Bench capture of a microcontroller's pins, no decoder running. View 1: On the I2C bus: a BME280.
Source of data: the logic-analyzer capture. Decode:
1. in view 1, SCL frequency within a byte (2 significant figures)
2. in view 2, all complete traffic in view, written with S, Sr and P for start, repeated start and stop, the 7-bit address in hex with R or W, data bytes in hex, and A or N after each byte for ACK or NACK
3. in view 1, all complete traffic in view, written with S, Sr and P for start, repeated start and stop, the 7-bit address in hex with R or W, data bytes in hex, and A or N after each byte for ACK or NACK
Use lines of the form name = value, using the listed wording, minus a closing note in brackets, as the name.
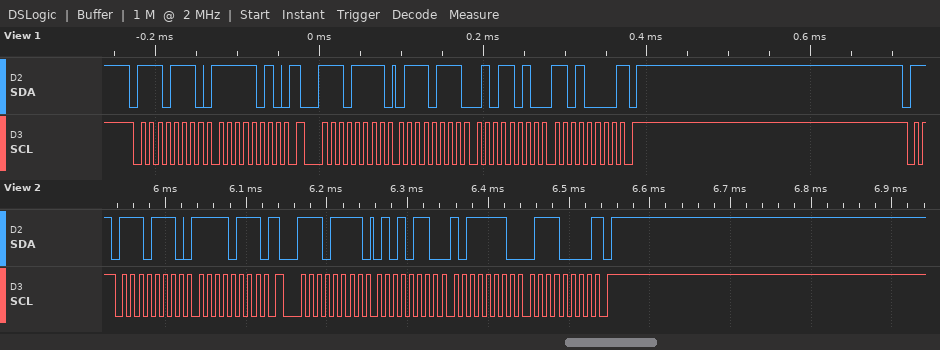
in view 1, SCL frequency within a byte = 100 kHz
in view 2, all complete traffic in view, written with S, Sr and P for start, repeated start and stop, the 7-bit address in hex with R or W, data bytes in hex, and A or N after each byte for ACK or NACK = S 77W A F7 A Sr 77R A 56 A BE A 70 N P
in view 1, all complete traffic in view, written with S, Sr and P for start, repeated start and stop, the 7-bit address in hex with R or W, data bytes in hex, and A or N after each byte for ACK or NACK = S 77W A FA A Sr 77R A 77 A 5A A D0 N P
